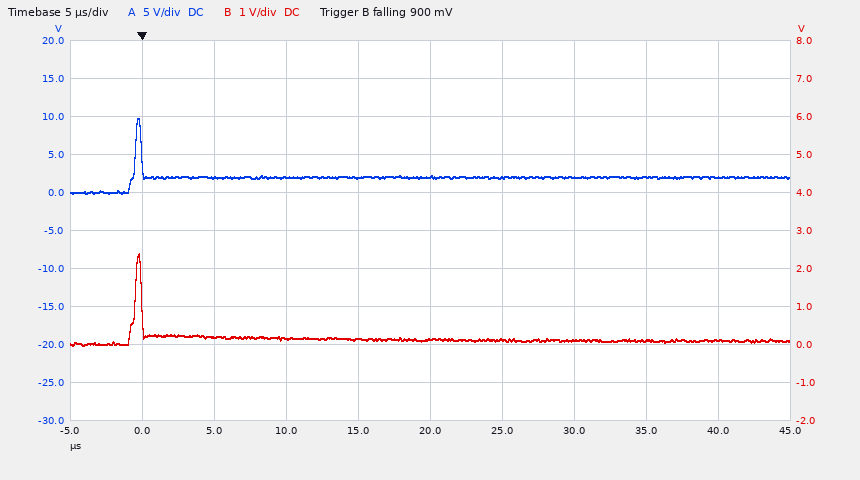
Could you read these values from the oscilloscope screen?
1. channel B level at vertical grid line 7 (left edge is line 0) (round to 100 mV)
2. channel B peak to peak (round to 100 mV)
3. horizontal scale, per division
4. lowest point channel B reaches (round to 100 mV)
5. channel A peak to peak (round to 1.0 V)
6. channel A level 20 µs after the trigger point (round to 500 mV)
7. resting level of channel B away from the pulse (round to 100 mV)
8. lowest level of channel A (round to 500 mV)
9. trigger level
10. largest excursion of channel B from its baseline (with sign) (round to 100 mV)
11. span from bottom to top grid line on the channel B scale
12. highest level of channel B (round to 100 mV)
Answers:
100 mV
2.4 V
5 µs
0.0 V
10.0 V
2.0 V
100 mV
0.0 V
900 mV
+2.3 V
10 V
2.4 V
